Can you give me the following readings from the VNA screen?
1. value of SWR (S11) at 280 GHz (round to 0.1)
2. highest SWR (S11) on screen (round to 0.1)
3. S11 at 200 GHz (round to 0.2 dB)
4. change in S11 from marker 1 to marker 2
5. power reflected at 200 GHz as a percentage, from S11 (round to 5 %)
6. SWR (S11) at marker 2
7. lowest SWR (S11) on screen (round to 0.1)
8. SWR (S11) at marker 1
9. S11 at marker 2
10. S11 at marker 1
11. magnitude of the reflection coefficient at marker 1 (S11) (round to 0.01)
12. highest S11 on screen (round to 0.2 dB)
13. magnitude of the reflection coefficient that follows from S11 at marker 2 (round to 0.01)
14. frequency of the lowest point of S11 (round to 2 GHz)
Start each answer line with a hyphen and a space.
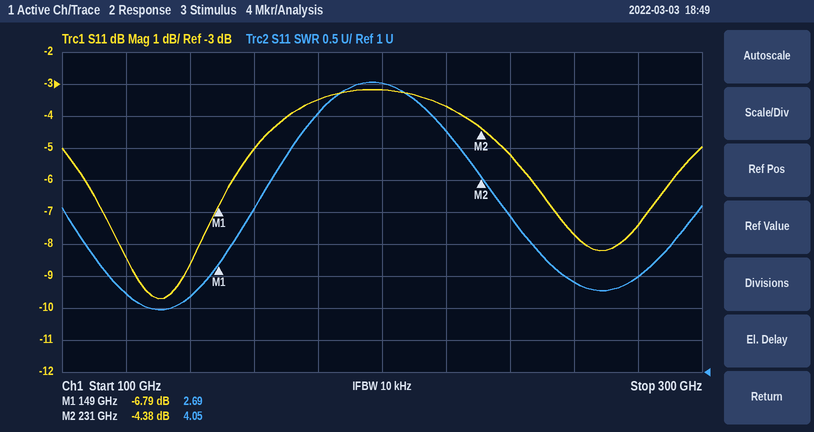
- 2.5
- 5.5
- -3.2 dB
- 2.41 dB
- 50 %
- 4.05
- 2.0
- 2.69
- -4.38 dB
- -6.79 dB
- 0.46
- -3.2 dB
- 0.60
- 130 GHz
